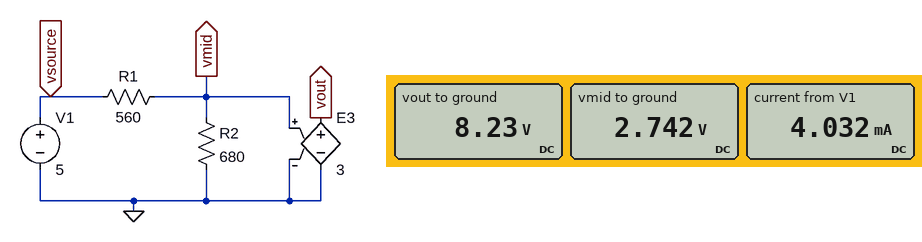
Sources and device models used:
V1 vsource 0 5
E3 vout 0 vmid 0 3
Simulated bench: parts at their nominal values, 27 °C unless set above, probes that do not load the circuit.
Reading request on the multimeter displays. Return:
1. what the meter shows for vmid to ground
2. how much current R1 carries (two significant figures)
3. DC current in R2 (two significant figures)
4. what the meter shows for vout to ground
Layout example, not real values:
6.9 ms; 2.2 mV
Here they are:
2.742 V; 4.0 mA; 4.0 mA; 8.23 V
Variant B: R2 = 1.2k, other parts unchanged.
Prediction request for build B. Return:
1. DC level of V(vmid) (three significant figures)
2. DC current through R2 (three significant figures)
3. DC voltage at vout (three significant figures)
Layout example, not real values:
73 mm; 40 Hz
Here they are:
3.41 V; 2.84 mA; 10.2 V
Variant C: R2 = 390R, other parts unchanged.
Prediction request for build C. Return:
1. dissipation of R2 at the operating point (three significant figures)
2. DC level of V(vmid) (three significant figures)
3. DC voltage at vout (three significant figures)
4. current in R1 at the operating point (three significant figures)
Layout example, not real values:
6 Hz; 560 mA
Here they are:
10.8 mW; 2.05 V; 6.16 V; 5.26 mA
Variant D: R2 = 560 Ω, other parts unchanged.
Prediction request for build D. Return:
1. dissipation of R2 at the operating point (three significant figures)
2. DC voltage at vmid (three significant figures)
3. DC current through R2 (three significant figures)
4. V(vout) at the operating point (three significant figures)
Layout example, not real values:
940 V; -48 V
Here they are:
11.2 mW; 2.50 V; 4.46 mA; 7.50 V
